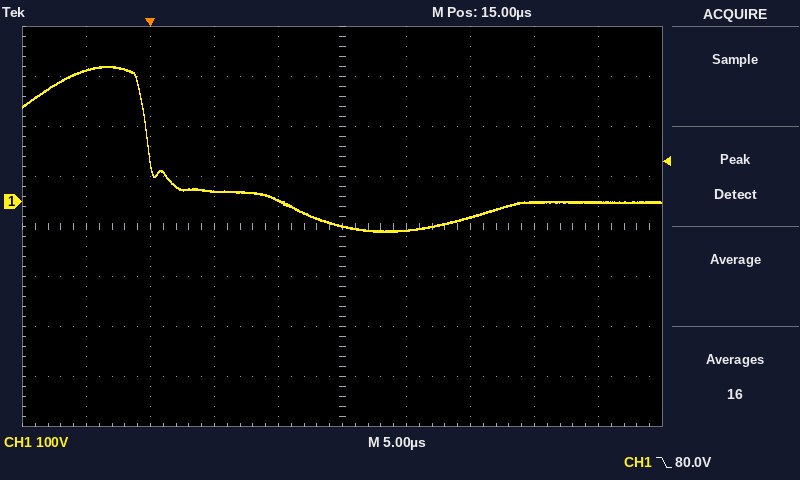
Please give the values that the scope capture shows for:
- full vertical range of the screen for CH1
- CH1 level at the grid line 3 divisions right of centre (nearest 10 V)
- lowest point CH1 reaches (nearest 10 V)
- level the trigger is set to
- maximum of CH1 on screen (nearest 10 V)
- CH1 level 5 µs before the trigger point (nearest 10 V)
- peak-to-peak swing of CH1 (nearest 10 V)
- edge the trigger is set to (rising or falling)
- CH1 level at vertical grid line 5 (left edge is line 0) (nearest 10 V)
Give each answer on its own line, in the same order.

800 V
0 V
-60 V
80.0 V
270 V
260 V
330 V
falling
-50 V
